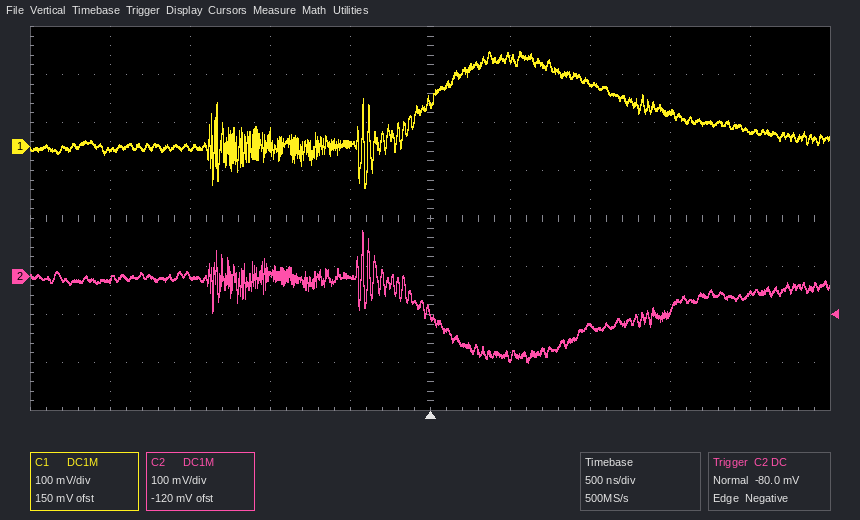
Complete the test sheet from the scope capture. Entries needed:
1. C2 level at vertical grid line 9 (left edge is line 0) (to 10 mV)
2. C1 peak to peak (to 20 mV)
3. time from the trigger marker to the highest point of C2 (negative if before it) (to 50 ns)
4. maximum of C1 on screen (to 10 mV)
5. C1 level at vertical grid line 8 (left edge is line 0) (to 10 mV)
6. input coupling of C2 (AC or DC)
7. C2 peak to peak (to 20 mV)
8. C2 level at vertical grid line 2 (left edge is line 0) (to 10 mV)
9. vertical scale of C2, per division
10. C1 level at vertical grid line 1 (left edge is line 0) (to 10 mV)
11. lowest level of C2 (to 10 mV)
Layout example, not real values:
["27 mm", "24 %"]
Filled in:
["-40 mV", "280 mV", "-400 ns", "200 mV", "70 mV", "DC", "280 mV", "0 mV", "100 mV", "-10 mV", "-180 mV"]
